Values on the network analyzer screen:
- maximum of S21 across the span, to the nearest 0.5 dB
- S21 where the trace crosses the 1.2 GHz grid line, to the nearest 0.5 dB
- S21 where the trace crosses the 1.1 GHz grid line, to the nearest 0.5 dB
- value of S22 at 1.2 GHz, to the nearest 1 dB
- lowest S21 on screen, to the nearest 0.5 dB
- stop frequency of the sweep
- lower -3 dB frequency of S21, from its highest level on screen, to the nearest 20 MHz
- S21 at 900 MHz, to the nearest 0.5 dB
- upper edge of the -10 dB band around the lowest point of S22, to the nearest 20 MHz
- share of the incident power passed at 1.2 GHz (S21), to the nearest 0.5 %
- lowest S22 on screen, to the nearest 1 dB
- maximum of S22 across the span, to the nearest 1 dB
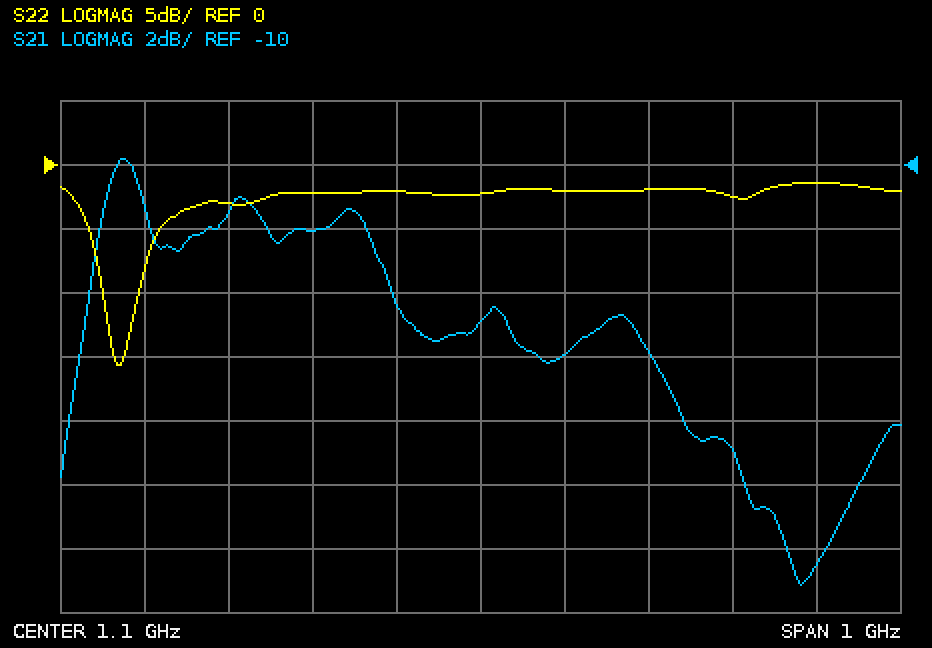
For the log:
-10.0 dB
-16.0 dB
-15.0 dB
-2 dB
-23.0 dB
1.6 GHz
640 MHz
-12.0 dB
700 MHz
2.5 %
-16 dB
-1 dB
